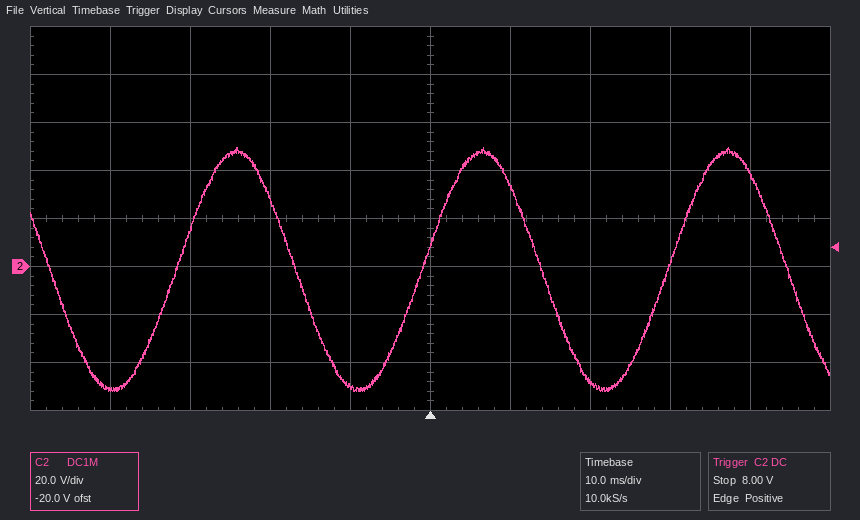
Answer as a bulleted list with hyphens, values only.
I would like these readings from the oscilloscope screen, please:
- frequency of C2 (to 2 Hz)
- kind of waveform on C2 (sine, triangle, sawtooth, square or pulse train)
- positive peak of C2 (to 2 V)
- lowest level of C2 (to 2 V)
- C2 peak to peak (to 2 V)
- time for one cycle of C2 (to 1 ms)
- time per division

- 32 Hz
- sine
- 50 V
- -52 V
- 102 V
- 31 ms
- 10 ms
